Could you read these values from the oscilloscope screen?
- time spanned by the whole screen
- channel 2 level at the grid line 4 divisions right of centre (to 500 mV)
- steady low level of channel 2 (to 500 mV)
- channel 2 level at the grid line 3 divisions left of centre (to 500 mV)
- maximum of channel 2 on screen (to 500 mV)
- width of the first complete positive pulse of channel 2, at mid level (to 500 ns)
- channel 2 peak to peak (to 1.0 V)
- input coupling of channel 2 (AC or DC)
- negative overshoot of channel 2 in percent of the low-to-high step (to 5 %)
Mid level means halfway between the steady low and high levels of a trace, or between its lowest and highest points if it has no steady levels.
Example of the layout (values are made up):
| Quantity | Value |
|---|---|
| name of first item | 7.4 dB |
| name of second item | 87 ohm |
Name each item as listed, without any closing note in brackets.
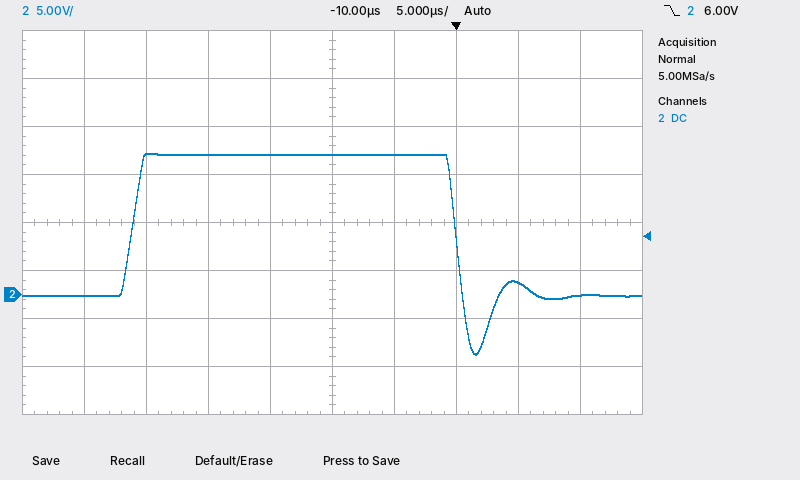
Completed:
| Quantity | Value |
|---|---|
| time spanned by the whole screen | 50 µs |
| channel 2 level at the grid line 4 divisions right of centre | 0.0 V |
| steady low level of channel 2 | 0.0 V |
| channel 2 level at the grid line 3 divisions left of centre | 14.5 V |
| maximum of channel 2 on screen | 14.5 V |
| width of the first complete positive pulse of channel 2, at mid level | 26.0 µs |
| channel 2 peak to peak | 21.0 V |
| input coupling of channel 2 | DC |
| negative overshoot of channel 2 in percent of the low-to-high step | 40 % |
